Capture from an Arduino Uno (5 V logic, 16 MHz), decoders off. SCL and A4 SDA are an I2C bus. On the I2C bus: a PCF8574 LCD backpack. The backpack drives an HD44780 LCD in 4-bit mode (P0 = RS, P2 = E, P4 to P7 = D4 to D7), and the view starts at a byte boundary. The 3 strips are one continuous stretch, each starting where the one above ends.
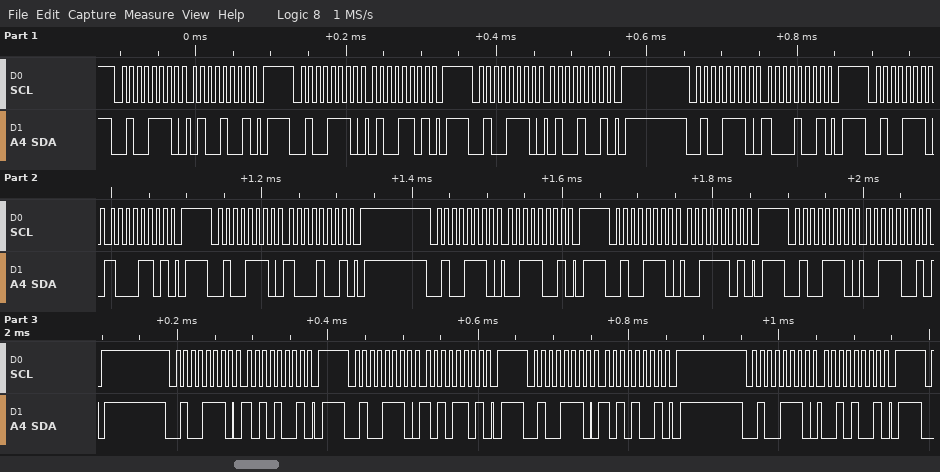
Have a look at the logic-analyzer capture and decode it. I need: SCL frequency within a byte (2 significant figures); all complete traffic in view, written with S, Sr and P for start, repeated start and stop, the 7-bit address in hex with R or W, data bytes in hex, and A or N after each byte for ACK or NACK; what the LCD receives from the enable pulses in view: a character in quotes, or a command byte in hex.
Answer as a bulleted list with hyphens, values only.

- 100 kHz
- S 27W A 49 A P S 27W A 4D A P S 27W A 49 A P S 27W A 89 A P S 27W A 8D A P S 27W A 89 A P S 27W A 39 A P S 27W A 3D A P S 27W A 39 A P S 27W A A9 A P S 27W A AD A P S 27W A A9 A P S 27W A 29 A P
- 'H' ':'
